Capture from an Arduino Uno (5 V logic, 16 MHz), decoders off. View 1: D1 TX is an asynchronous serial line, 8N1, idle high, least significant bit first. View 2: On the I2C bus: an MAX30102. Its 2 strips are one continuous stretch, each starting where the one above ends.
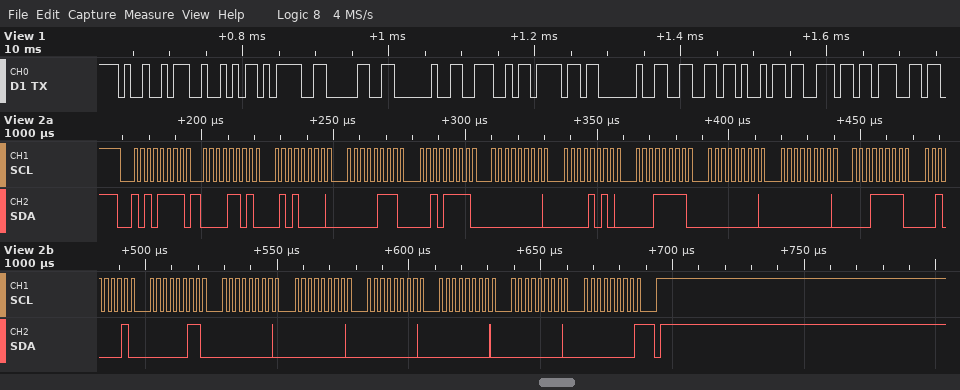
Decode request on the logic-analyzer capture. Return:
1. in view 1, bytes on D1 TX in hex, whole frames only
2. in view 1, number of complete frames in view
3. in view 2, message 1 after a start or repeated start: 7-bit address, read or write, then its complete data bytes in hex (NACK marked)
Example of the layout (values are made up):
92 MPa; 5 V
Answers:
49 52 3D 30 20 4E 6F 20 66 69 6E 67; 12; 0x57 read: 0D 50 07 2F 00 0A 1F 00 00 1F 21 03 00 00 00 00 00 00 NACK
